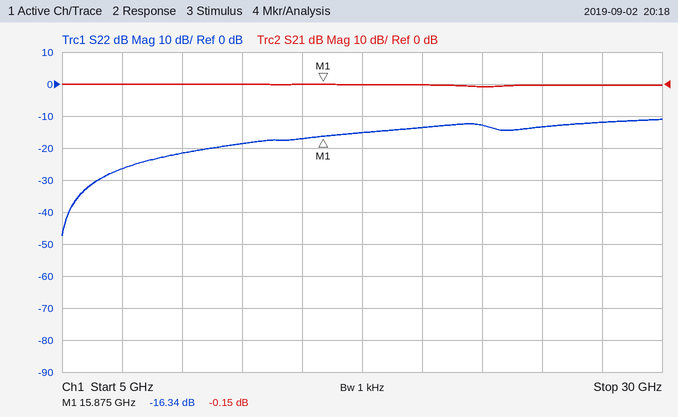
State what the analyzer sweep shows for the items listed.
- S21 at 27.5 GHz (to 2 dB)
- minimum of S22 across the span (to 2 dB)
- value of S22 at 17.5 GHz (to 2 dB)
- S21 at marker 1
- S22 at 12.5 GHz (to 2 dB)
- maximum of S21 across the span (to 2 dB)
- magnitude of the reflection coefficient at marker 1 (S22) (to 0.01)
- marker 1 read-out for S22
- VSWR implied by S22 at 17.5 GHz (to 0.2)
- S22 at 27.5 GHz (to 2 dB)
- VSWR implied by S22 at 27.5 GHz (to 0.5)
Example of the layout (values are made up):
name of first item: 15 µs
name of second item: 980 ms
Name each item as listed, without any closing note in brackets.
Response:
S21 at 27.5 GHz: 0 dB
minimum of S22 across the span: -48 dB
value of S22 at 17.5 GHz: -16 dB
S21 at marker 1: -0.15 dB
S22 at 12.5 GHz: -18 dB
maximum of S21 across the span: 0 dB
magnitude of the reflection coefficient at marker 1 (S22): 0.15
marker 1 read-out for S22: -16.34 dB
VSWR implied by S22 at 17.5 GHz: 1.4
S22 at 27.5 GHz: -12 dB
VSWR implied by S22 at 27.5 GHz: 1.5
